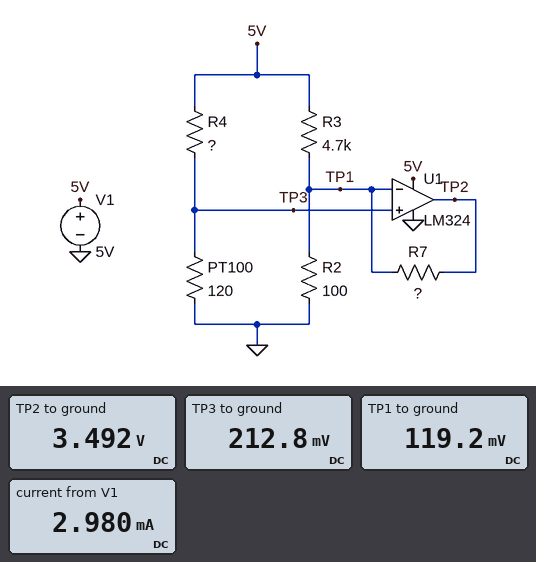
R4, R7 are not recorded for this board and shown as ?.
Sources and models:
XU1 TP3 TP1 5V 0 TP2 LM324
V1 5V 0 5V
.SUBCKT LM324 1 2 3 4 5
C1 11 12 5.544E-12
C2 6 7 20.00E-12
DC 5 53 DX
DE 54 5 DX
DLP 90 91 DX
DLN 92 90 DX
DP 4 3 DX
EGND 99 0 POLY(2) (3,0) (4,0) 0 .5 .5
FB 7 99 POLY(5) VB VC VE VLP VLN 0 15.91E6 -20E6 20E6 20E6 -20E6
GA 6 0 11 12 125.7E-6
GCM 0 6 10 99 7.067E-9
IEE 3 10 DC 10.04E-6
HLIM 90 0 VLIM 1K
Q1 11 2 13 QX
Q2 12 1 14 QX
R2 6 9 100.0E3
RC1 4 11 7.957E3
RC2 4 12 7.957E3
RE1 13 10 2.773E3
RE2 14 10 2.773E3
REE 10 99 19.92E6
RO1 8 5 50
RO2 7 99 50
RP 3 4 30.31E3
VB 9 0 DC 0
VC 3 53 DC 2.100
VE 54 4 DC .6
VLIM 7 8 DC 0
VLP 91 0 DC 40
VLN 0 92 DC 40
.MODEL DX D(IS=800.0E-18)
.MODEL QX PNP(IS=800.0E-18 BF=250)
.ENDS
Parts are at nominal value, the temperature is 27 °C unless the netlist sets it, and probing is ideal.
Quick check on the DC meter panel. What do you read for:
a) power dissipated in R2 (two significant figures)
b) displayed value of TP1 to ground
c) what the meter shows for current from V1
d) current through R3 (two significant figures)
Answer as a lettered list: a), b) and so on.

a) 140 µW
b) 119.2 mV
c) 2.980 mA
d) 1.0 mA
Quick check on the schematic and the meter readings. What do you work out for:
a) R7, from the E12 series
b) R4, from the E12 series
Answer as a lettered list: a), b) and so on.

a) 22 kΩ
b) 2.7 kΩ
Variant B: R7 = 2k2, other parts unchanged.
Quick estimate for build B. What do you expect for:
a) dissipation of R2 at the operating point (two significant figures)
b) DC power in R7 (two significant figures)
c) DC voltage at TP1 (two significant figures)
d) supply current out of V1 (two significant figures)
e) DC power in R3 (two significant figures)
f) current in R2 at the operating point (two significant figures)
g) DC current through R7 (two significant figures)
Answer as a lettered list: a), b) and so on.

a) 450 µW
b) 2.7 mW
c) 210 mV
d) 3.0 mA
e) 4.9 mW
f) 2.1 mA
g) 1.1 mA
